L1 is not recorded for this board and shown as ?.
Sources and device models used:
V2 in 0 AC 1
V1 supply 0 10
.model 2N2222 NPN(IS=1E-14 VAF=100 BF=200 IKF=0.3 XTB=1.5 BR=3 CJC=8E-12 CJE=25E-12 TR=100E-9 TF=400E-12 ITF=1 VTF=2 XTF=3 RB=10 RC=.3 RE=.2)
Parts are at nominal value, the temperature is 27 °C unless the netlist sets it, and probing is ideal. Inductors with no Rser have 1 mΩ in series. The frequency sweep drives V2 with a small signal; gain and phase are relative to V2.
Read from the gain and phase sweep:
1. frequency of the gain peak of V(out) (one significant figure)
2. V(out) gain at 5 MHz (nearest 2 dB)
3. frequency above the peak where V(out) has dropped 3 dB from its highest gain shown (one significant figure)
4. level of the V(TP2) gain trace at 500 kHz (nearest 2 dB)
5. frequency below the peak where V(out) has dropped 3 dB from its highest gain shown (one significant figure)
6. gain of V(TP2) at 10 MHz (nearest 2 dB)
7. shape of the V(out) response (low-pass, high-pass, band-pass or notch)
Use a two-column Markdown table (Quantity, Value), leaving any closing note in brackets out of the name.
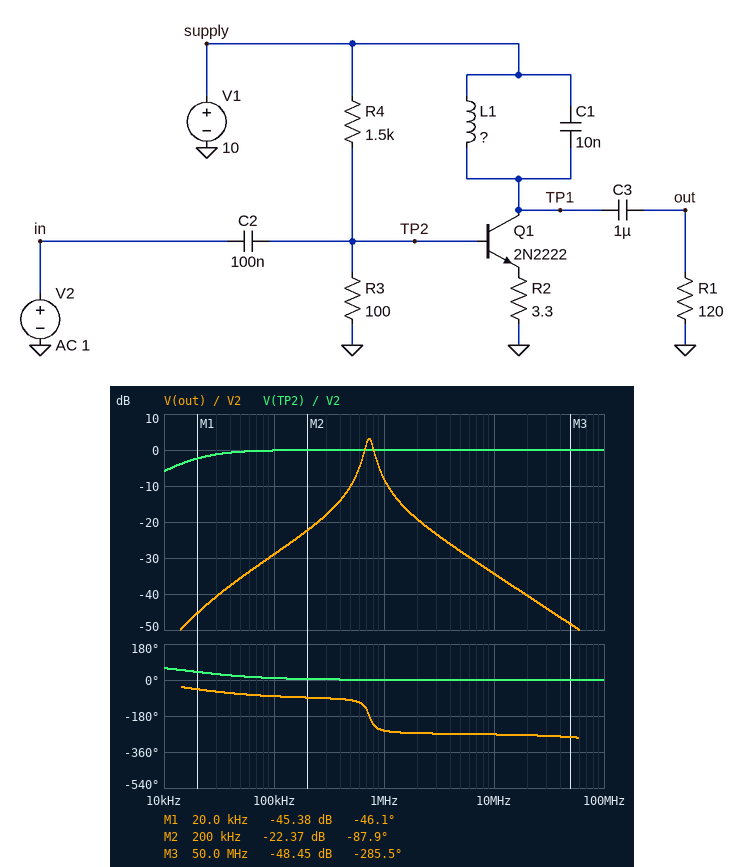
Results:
| Quantity | Value |
|---|---|
| frequency of the gain peak of V(out) | 700 kHz |
| V(out) gain at 5 MHz | -28 dB |
| frequency above the peak where V(out) has dropped 3 dB from its highest gain shown | 800 kHz |
| level of the V(TP2) gain trace at 500 kHz | 0 dB |
| frequency below the peak where V(out) has dropped 3 dB from its highest gain shown | 700 kHz |
| gain of V(TP2) at 10 MHz | 0 dB |
| shape of the V(out) response | band-pass |
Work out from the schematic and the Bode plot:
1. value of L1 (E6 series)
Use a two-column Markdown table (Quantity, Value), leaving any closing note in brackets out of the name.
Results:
| Quantity | Value |
|---|---|
| value of L1 | 4.7 µH |
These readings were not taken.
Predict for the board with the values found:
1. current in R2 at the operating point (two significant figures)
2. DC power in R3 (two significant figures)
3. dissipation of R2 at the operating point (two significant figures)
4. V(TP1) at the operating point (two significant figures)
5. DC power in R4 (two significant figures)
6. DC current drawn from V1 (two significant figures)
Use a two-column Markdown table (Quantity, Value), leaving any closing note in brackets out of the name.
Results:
| Quantity | Value |
|---|---|
| current in R2 at the operating point | 330 µA |
| DC power in R3 | 3.9 mW |
| dissipation of R2 at the operating point | 350 nW |
| V(TP1) at the operating point | 10 V |
| DC power in R4 | 59 mW |
| DC current drawn from V1 | 6.6 mA |
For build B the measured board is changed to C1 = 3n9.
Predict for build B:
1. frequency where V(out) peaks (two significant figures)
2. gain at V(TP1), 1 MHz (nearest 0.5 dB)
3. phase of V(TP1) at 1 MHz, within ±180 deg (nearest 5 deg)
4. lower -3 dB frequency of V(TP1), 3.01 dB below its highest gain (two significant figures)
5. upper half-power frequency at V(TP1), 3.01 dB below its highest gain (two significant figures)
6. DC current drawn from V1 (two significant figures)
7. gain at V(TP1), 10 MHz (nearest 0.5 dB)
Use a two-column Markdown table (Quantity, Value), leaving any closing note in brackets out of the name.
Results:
| Quantity | Value |
|---|---|
| frequency where V(out) peaks | 1.2 MHz |
| gain at V(TP1), 1 MHz | -0.5 dB |
| phase of V(TP1) at 1 MHz, within ±180 deg | -130 deg |
| lower -3 dB frequency of V(TP1), 3.01 dB below its highest gain | 1.0 MHz |
| upper half-power frequency at V(TP1), 3.01 dB below its highest gain | 1.4 MHz |
| DC current drawn from V1 | 6.6 mA |
| gain at V(TP1), 10 MHz | -26.0 dB |
